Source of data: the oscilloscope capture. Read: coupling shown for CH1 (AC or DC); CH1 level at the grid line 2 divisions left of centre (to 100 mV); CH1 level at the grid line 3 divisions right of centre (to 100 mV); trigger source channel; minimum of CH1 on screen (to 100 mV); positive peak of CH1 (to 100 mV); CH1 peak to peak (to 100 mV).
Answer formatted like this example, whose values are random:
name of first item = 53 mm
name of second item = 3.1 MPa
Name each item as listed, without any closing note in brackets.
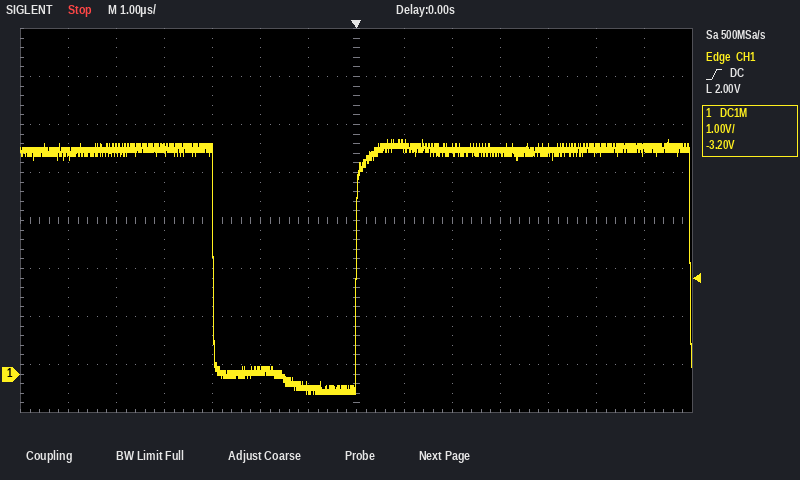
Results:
coupling shown for CH1 = DC
CH1 level at the grid line 2 divisions left of centre = 100 mV
CH1 level at the grid line 3 divisions right of centre = 4.6 V
trigger source channel = CH1
minimum of CH1 on screen = -400 mV
positive peak of CH1 = 4.9 V
CH1 peak to peak = 5.3 V
